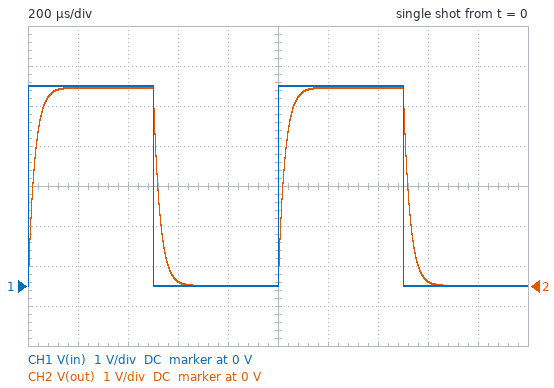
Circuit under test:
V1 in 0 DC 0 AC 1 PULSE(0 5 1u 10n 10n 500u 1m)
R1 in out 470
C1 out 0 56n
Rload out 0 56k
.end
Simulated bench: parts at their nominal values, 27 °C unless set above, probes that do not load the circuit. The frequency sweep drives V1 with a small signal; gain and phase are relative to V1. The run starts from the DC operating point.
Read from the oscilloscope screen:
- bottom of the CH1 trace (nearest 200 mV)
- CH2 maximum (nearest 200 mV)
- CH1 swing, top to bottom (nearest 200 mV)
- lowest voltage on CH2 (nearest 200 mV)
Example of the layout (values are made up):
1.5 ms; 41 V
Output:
0 V; 5.0 V; 5.0 V; 0 V
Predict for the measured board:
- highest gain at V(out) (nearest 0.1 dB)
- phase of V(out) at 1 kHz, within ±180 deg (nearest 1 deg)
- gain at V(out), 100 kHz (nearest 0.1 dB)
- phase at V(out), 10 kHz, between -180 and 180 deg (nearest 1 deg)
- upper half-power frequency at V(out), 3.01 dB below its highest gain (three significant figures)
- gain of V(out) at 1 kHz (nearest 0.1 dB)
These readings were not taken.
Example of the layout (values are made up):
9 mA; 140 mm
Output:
-0.1 dB; -9 deg; -24.4 dB; -59 deg; 6.10 kHz; -0.2 dB
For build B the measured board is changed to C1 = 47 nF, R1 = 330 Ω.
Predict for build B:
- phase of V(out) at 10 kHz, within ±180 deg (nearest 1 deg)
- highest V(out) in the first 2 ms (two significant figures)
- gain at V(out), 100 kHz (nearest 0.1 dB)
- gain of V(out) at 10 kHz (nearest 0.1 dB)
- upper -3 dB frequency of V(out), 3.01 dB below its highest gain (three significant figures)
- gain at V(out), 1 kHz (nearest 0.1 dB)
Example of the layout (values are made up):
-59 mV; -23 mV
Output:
-44 deg; 5.0 V; -19.8 dB; -2.9 dB; 10.3 kHz; -0.1 dB
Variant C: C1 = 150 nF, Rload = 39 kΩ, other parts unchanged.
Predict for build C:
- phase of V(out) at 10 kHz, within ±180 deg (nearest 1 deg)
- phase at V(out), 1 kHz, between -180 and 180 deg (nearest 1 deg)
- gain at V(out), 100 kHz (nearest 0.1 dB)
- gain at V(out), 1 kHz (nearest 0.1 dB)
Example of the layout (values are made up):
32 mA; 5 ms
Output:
-77 deg; -24 deg; -32.9 dB; -0.9 dB
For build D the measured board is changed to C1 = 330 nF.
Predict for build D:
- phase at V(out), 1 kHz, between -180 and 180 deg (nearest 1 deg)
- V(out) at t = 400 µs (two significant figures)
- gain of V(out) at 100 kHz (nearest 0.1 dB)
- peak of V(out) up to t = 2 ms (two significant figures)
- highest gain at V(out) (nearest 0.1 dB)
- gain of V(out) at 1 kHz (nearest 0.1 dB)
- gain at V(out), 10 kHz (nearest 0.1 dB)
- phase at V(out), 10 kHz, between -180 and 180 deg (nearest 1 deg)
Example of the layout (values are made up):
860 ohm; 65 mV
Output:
-44 deg; 4.6 V; -39.8 dB; 4.8 V; -0.1 dB; -2.9 dB; -19.8 dB; -84 deg
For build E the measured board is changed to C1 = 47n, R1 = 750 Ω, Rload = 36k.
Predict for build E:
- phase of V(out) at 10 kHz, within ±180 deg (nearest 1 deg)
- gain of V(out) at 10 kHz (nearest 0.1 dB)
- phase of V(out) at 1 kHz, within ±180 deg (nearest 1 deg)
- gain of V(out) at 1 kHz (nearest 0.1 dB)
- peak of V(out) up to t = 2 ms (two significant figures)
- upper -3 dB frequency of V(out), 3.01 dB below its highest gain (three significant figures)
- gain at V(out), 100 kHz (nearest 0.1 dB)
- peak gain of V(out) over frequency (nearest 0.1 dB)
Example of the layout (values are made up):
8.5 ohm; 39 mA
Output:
-65 deg; -7.7 dB; -12 deg; -0.4 dB; 4.9 V; 4.61 kHz; -26.9 dB; -0.2 dB
